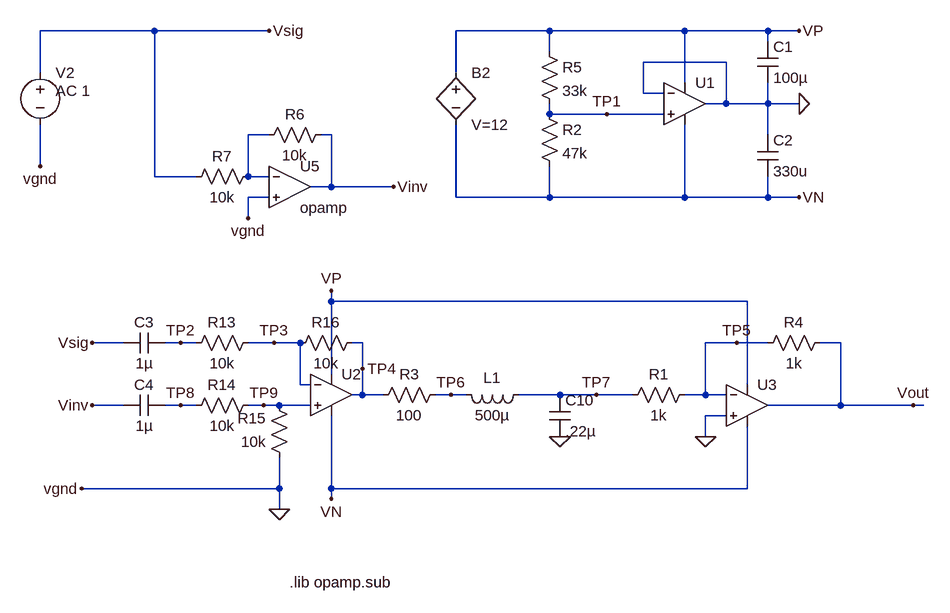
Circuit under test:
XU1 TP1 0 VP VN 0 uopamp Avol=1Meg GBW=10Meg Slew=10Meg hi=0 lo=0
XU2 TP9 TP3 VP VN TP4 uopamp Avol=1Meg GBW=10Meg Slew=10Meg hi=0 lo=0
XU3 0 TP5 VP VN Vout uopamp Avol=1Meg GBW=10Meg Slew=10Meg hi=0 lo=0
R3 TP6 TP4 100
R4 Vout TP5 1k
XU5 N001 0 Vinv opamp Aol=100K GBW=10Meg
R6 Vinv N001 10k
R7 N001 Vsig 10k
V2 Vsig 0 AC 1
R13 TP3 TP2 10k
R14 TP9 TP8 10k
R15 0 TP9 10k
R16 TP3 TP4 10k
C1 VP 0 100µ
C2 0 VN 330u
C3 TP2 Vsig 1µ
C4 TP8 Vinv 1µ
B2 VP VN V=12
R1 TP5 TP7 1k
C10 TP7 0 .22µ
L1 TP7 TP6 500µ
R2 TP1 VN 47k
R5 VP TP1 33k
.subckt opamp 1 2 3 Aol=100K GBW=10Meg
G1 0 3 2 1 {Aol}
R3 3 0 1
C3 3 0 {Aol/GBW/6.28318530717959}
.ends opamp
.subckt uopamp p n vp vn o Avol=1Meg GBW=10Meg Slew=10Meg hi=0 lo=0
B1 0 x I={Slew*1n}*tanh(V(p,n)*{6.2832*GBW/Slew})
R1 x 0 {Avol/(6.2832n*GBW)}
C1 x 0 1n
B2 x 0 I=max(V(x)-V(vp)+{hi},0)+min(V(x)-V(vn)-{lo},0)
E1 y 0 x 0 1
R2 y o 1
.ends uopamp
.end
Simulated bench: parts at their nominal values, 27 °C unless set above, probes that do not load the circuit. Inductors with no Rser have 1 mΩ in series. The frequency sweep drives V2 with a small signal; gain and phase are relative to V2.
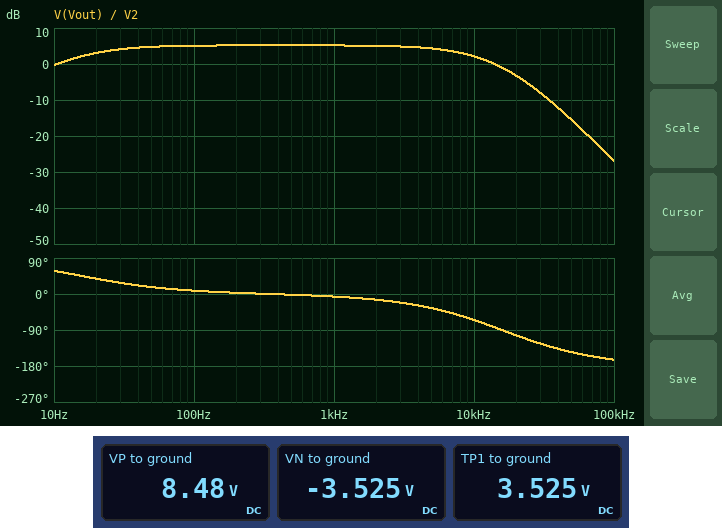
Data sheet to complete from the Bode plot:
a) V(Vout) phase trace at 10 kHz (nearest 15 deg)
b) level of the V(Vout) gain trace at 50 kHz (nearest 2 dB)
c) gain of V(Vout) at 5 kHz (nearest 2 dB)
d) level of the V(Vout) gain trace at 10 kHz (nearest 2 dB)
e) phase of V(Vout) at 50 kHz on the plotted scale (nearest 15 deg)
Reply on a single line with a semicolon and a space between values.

-60 deg; -16 dB; 4 dB; 2 dB; -150 deg
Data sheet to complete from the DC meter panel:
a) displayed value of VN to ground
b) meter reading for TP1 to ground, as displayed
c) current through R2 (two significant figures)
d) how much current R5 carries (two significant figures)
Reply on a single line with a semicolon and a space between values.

-3.525 V; 3.525 V; 150 µA; 150 µA
